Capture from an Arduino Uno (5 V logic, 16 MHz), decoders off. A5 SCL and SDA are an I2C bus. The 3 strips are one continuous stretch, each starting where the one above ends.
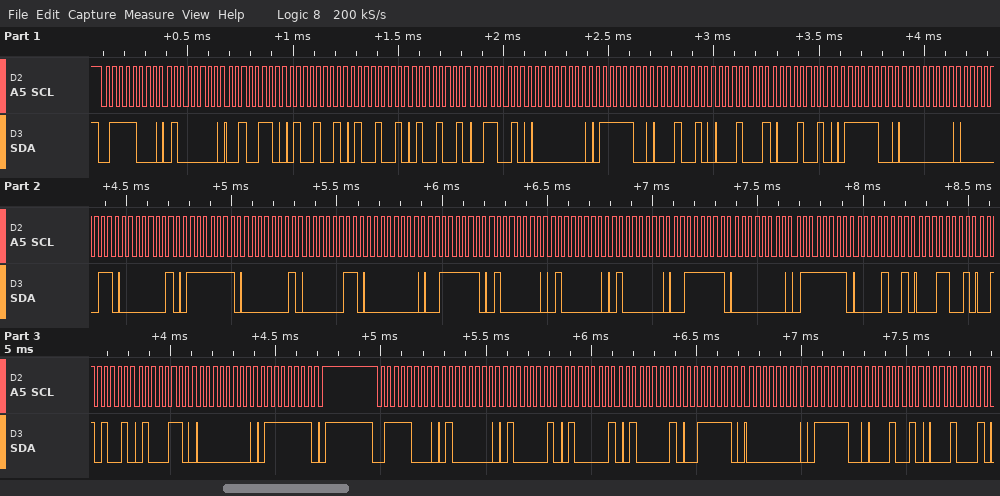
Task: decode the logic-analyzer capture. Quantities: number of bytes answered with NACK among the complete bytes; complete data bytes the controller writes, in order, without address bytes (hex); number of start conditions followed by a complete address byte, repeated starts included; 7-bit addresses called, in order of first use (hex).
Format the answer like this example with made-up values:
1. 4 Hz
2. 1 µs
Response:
1. 0
2. 40 26 49 49 49 32 00 7C 12 11 12 7C 00 03 01 7F 01 03 00 3F 40 40 40 3F 00 7F 09 19 29 46 00 7F 40 41 41 41 3E 00 7C 12 11
3. 2
4. 0x3C
